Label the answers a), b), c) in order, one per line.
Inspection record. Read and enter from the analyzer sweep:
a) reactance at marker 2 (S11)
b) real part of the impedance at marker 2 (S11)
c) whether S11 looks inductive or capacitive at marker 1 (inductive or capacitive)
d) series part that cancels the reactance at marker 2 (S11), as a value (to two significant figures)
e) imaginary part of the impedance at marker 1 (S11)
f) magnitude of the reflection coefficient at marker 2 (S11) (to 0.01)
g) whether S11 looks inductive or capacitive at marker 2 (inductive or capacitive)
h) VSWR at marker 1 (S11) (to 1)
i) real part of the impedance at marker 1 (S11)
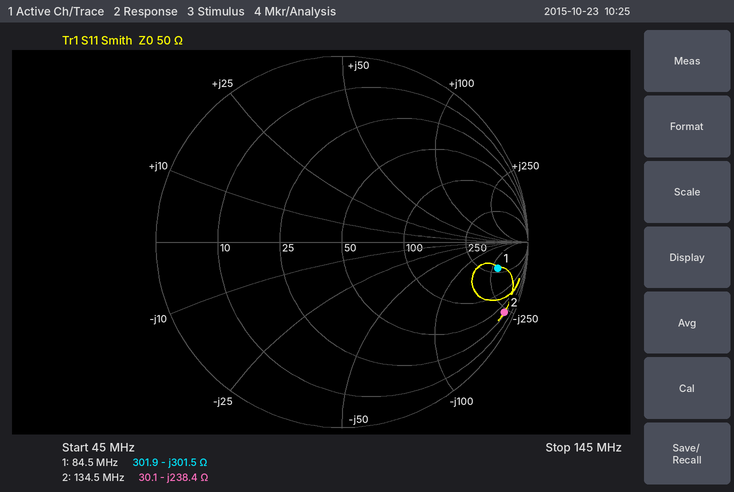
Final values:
a) -238.4 Ω
b) 30.1 Ω
c) capacitive
d) 280 nH
e) -301.5 Ω
f) 0.95
g) capacitive
h) 12
i) 301.9 Ω
